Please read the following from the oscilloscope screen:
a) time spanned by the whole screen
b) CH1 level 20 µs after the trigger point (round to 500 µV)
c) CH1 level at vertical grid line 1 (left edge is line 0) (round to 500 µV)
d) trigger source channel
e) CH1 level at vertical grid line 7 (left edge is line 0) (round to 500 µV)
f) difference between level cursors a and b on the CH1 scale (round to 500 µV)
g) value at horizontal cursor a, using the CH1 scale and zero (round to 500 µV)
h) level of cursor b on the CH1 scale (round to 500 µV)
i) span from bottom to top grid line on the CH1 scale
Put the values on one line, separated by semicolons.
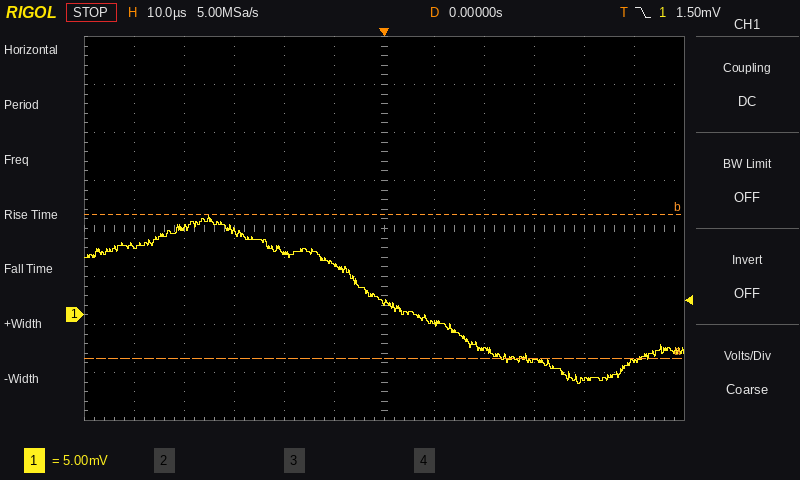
120 µs; -3.5 mV; 7.0 mV; CH1; -1.0 mV; 15.0 mV; -4.5 mV; 10.5 mV; 40 mV
